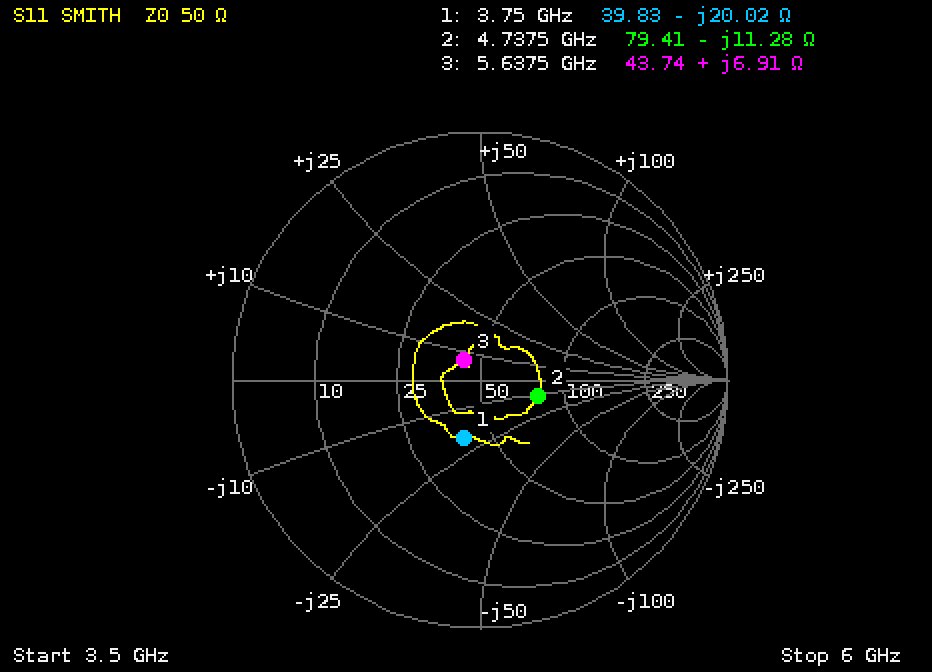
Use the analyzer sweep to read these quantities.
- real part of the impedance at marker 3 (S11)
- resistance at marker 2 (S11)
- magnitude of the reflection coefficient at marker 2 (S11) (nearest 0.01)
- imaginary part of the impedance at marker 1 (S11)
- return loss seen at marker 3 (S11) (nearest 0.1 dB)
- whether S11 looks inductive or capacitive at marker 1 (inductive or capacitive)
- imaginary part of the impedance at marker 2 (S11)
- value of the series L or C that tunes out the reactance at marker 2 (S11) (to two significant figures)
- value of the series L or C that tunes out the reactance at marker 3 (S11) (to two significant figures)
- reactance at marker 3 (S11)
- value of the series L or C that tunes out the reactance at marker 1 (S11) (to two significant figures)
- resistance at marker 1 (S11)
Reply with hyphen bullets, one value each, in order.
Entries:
- 43.74 Ω
- 79.41 Ω
- 0.24
- -20.02 Ω
- 20.1 dB
- capacitive
- -11.28 Ω
- 380 pH
- 4.1 pF
- +6.91 Ω
- 850 pH
- 39.83 Ω
